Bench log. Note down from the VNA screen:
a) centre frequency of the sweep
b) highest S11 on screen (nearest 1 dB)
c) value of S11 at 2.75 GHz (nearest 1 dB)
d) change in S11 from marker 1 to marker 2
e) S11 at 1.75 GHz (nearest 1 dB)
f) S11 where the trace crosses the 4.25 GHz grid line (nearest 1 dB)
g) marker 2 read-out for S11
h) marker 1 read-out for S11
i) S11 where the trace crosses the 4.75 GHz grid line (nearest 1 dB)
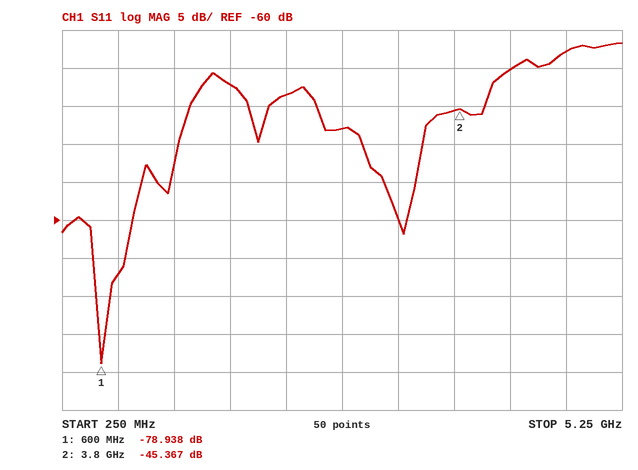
2.75 GHz
-37 dB
-48 dB
33.571 dB
-42 dB
-40 dB
-45.367 dB
-78.938 dB
-38 dB
